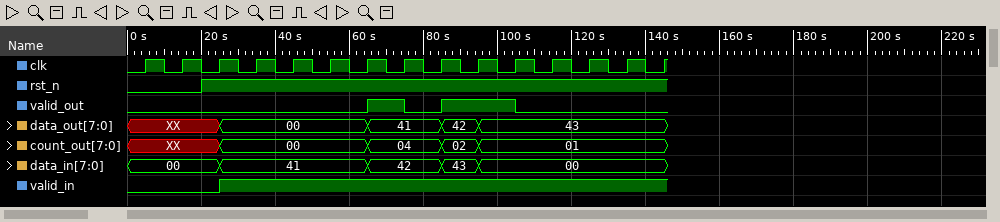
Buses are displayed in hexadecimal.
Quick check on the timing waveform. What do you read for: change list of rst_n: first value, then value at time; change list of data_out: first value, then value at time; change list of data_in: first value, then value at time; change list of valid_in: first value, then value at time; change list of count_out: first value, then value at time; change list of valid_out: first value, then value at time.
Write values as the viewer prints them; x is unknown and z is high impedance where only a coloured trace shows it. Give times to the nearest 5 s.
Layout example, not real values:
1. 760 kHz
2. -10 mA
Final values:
1. 0, 1 at 20 s
2. XX, 00 at 25 s, 41 at 65 s, 42 at 85 s, 43 at 95 s
3. 00, 41 at 25 s, 42 at 65 s, 43 at 85 s, 00 at 95 s
4. 0, 1 at 25 s
5. XX, 00 at 25 s, 04 at 65 s, 02 at 85 s, 01 at 95 s
6. 0, 1 at 65 s, 0 at 75 s, 1 at 85 s, 0 at 105 s
